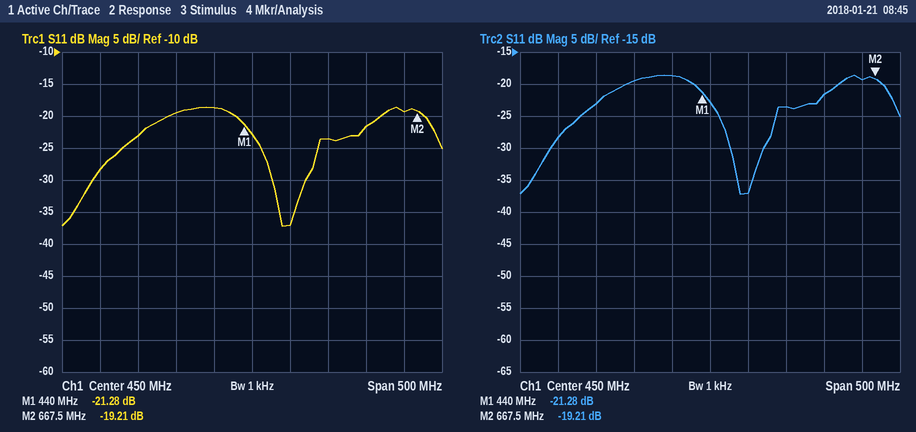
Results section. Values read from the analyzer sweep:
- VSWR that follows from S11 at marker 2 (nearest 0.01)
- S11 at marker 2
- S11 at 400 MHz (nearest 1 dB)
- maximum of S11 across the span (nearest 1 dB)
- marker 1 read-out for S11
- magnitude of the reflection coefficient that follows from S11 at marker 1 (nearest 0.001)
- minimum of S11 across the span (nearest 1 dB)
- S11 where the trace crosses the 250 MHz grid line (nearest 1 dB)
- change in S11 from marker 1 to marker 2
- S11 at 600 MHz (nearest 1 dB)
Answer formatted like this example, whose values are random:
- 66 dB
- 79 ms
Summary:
- 1.25
- -19.21 dB
- -19 dB
- -19 dB
- -21.28 dB
- 0.086
- -37 dB
- -28 dB
- 2.07 dB
- -22 dB
